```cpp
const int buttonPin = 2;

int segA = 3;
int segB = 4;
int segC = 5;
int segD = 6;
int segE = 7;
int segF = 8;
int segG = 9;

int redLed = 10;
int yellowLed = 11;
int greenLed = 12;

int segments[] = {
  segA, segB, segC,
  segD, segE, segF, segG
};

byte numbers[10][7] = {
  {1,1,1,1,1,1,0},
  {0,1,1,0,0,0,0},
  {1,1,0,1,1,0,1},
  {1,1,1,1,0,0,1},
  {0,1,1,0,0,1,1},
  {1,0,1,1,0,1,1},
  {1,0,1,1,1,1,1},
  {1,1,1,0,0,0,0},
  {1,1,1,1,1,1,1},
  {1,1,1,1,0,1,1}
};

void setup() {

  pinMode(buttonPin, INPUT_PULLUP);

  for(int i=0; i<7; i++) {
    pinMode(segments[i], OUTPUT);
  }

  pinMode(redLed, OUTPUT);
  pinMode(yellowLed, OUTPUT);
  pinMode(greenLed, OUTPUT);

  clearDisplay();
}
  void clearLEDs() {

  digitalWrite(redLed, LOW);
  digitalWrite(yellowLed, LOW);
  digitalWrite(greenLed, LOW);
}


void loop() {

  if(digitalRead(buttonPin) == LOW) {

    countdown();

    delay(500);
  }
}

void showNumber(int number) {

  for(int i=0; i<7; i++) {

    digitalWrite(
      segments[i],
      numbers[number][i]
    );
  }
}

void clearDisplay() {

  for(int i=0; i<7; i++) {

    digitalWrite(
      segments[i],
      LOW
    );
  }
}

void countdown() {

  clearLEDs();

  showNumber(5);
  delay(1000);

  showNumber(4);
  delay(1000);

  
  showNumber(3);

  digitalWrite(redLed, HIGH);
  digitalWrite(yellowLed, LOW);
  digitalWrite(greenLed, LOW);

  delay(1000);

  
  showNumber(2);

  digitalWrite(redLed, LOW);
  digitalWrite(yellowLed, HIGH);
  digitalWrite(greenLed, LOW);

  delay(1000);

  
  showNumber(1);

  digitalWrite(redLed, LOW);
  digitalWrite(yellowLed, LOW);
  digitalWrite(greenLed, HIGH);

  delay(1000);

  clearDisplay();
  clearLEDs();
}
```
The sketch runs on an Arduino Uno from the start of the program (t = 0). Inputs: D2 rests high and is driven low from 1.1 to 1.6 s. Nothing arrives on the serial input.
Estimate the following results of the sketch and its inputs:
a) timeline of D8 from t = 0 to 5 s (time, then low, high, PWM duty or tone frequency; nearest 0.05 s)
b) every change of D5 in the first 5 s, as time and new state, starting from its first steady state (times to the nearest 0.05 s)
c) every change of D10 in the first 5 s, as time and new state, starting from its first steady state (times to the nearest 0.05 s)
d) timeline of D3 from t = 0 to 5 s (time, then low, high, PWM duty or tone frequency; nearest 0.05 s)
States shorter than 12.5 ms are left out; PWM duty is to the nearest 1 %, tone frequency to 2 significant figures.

0 s low; 1.1 s high; 3.1 s low
0 s low; 1.1 s high; 4.1 s low
0 s low; 3.1 s high; 4.1 s low
0 s low; 1.1 s high; 2.1 s low; 3.1 s high
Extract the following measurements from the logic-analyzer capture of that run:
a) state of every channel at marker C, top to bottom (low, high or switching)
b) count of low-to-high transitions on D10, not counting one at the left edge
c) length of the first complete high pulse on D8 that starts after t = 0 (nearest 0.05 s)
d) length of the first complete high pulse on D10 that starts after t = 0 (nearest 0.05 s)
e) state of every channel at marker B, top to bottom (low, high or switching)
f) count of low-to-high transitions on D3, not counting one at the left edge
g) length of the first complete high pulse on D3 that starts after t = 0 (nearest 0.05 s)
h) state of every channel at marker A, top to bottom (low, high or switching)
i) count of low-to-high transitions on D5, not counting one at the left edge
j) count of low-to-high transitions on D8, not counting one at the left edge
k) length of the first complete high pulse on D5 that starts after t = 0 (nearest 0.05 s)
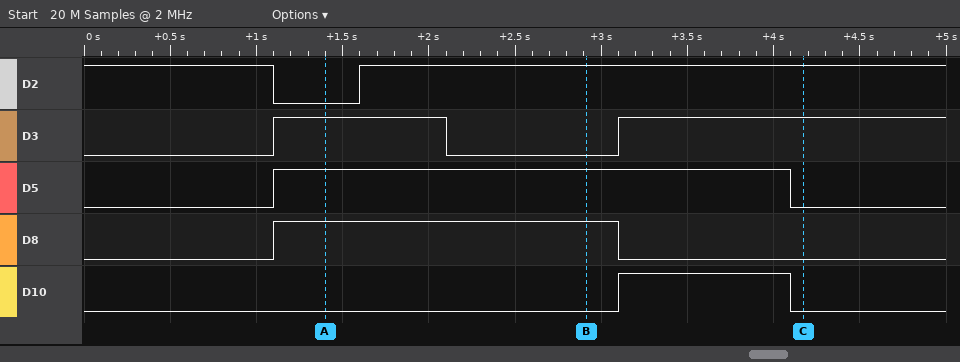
D2 high, D3 high, D5 low, D8 low, D10 low
1
2.00 s
1.00 s
D2 high, D3 low, D5 high, D8 high, D10 low
2
1.00 s
D2 low, D3 high, D5 high, D8 high, D10 low
1
1
3.00 s
